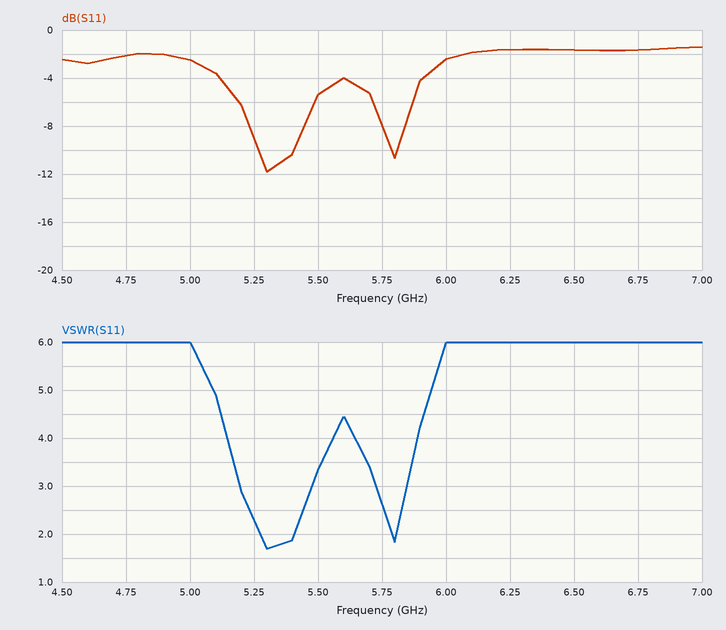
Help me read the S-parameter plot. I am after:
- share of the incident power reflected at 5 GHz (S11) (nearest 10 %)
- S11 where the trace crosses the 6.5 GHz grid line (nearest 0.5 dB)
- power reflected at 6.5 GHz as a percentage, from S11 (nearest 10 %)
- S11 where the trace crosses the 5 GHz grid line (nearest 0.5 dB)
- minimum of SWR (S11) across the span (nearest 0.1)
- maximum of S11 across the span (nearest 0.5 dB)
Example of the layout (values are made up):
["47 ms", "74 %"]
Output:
["60 %", "-1.5 dB", "70 %", "-2.5 dB", "1.7", "-1.5 dB"]
